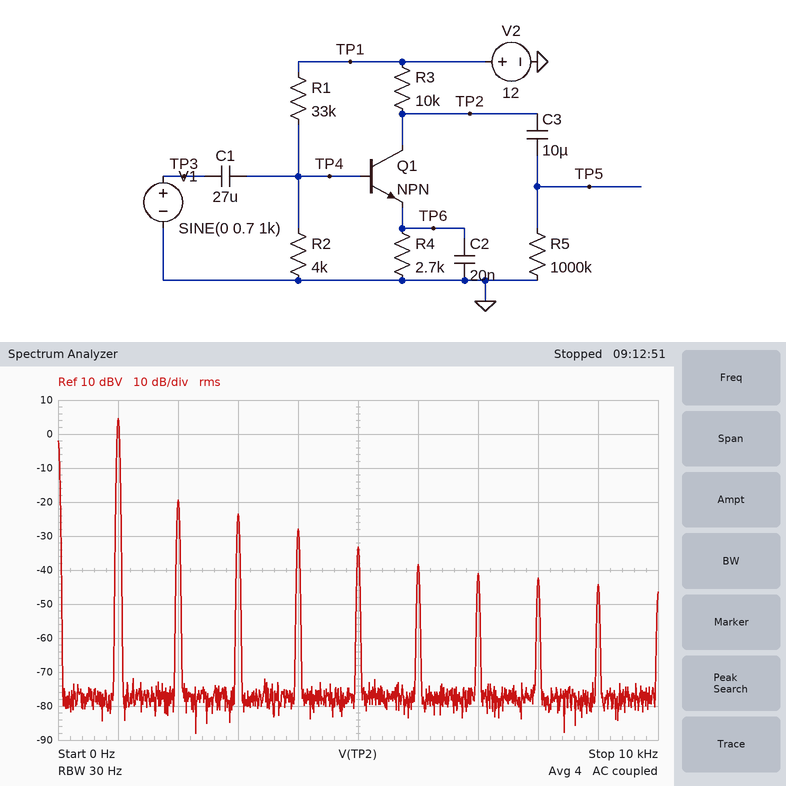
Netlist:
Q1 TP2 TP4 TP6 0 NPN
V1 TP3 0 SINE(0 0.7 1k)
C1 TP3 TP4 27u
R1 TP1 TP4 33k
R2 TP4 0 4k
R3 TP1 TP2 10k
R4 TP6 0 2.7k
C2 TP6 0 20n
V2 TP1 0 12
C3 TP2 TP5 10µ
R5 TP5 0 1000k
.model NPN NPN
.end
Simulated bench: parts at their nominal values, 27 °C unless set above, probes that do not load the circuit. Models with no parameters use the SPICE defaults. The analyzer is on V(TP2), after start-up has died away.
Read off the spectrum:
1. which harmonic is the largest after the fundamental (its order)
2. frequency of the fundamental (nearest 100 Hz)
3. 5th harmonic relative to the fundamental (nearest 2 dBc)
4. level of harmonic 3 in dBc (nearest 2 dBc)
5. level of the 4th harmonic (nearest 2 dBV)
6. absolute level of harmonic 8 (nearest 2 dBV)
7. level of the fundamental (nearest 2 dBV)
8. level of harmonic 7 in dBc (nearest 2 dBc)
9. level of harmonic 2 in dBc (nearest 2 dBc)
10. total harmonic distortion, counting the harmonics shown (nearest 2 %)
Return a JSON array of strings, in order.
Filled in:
["2", "1.0 kHz", "-38 dBc", "-28 dBc", "-28 dBV", "-42 dBV", "4 dBV", "-46 dBc", "-24 dBc", "8 %"]
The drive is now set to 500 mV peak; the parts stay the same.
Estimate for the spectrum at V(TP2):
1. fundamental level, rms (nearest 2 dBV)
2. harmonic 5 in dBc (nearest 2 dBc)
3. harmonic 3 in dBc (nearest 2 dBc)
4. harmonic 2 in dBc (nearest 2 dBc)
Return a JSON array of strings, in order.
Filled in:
["2 dBV", "-56 dBc", "-42 dBc", "-34 dBc"]
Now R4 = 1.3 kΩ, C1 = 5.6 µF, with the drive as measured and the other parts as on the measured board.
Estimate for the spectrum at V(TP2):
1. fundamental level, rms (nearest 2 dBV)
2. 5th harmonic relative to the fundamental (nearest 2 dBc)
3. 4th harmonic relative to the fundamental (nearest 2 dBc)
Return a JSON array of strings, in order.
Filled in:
["10 dBV", "-40 dBc", "-34 dBc"]
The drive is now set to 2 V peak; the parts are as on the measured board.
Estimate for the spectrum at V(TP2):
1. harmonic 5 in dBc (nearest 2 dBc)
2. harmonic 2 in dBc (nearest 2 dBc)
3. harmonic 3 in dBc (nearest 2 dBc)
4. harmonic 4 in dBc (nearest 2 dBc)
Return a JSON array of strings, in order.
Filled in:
["-28 dBc", "-10 dBc", "-22 dBc", "-26 dBc"]
